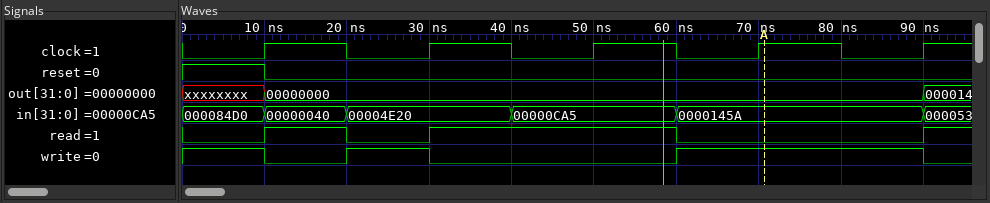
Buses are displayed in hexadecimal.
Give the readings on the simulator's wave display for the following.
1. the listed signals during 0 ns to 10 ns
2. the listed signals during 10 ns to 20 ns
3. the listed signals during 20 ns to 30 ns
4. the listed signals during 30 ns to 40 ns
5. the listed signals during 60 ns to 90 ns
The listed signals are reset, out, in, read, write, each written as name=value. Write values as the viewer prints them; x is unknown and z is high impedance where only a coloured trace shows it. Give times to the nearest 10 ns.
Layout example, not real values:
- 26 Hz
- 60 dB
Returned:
- reset=1, out=xxxxxxxx, in=000084D0, read=0, write=1
- reset=0, out=00000000, in=00000040, read=1, write=0
- reset=0, out=00000000, in=00004E20, read=0, write=1
- reset=0, out=00000000, in=00004E20, read=1, write=0
- reset=0, out=00000000, in=0000145A, read=0, write=1
